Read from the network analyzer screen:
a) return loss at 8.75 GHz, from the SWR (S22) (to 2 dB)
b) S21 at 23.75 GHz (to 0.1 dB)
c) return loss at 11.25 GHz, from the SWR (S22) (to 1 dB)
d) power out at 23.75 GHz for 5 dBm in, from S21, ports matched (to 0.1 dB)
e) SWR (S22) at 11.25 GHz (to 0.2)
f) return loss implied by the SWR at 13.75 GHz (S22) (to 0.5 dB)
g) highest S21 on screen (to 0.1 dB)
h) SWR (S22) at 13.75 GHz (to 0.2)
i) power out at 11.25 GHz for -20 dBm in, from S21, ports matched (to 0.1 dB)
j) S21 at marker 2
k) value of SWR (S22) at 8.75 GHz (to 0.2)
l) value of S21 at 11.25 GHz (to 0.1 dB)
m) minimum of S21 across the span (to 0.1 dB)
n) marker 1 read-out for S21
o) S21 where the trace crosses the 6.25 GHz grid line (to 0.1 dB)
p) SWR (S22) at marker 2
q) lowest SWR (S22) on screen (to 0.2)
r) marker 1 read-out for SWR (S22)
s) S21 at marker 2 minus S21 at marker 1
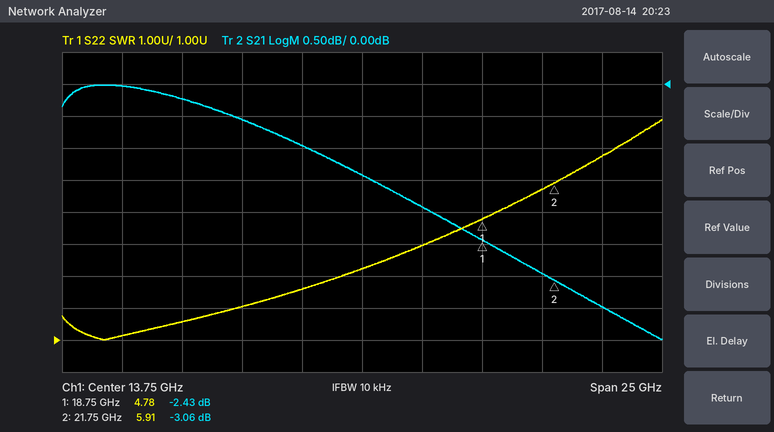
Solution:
10 dB
-3.5 dB
7 dB
1.5 dBm
2.6
5.5 dB
0.0 dB
3.2
-21.0 dBm
-3.06 dB
2.0
-1.0 dB
-4.0 dB
-2.43 dB
-0.2 dB
5.91
1.0
4.78
-0.63 dB
